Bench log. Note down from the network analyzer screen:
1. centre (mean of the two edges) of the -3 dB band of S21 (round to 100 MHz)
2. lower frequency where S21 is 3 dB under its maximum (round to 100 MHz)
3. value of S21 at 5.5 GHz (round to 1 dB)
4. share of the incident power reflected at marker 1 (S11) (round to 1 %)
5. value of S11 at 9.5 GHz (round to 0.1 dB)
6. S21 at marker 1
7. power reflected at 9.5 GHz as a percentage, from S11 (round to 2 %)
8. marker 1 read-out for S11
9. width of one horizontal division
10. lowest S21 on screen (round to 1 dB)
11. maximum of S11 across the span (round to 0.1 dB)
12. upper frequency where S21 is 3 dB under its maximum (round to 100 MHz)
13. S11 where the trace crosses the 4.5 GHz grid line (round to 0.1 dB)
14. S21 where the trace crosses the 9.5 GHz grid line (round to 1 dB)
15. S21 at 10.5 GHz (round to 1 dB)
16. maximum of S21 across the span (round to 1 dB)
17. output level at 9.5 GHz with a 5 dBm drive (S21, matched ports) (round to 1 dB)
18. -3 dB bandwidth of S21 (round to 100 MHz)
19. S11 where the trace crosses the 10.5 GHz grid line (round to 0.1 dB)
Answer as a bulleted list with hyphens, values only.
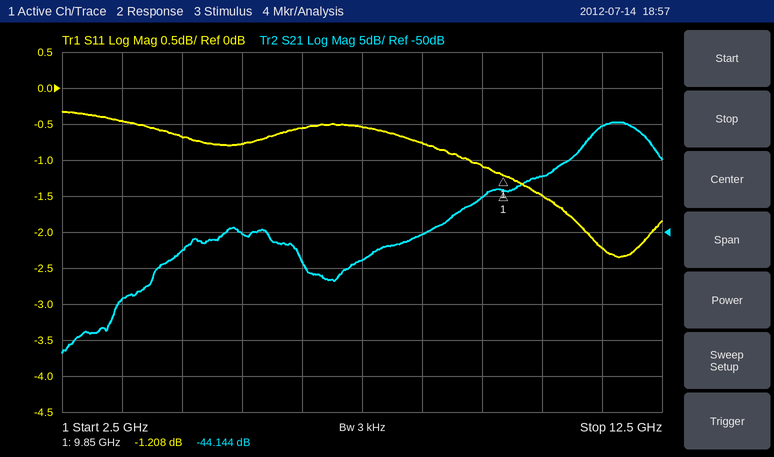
- 11.8 GHz
- 11.2 GHz
- -50 dB
- 76 %
- -1.1 dB
- -44.144 dB
- 78 %
- -1.208 dB
- 1 GHz
- -67 dB
- -0.3 dB
- 12.3 GHz
- -0.7 dB
- -45 dB
- -42 dB
- -35 dB
- -40 dBm
- 1.1 GHz
- -1.5 dB
